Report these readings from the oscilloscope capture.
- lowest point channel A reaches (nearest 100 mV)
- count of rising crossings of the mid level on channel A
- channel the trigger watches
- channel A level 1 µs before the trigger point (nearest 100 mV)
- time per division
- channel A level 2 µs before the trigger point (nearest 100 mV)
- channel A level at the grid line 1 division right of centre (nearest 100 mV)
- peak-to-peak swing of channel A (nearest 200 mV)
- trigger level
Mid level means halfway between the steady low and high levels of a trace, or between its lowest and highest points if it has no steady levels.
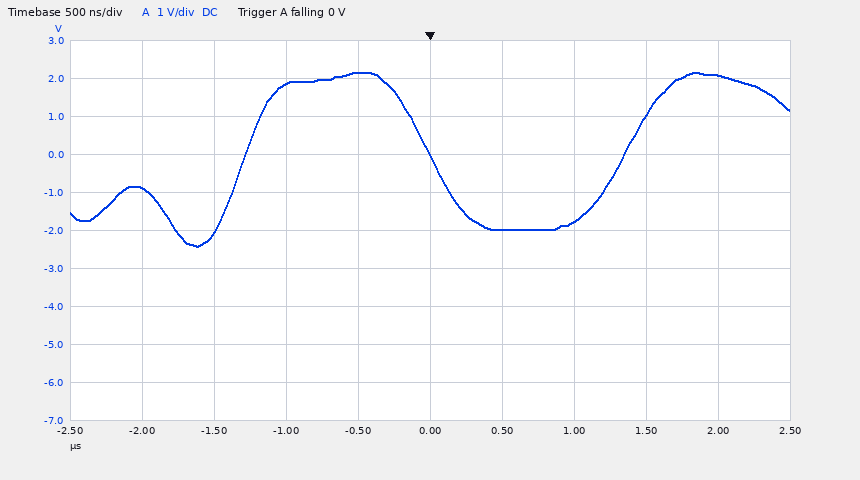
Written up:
-2.4 V
2
channel A
1.9 V
500 ns
-900 mV
-2.0 V
4.6 V
0 V
